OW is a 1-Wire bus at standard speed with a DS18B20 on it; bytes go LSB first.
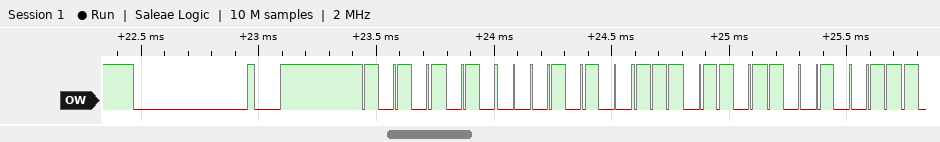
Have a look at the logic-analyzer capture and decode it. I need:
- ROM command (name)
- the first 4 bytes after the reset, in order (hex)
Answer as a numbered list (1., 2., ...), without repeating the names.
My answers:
1. Match ROM
2. 55 28 B7 C9
